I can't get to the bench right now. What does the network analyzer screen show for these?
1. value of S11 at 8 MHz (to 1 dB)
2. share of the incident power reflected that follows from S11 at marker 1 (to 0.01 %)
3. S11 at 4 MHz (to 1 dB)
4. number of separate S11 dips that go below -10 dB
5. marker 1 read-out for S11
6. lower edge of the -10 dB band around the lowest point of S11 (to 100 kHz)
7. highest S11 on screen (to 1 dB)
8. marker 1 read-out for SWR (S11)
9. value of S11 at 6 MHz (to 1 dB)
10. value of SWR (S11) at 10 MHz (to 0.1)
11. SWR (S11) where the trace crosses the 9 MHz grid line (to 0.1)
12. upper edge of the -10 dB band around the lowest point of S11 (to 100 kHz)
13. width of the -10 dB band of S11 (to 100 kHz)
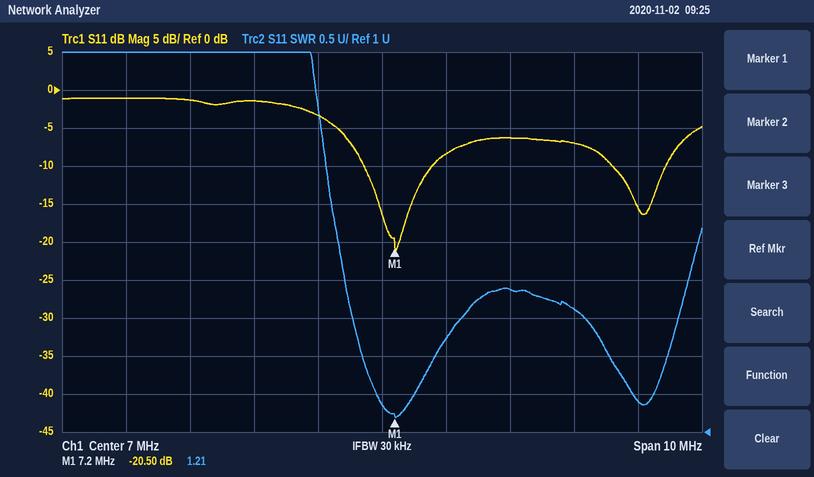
-8 dB
0.89 %
-1 dB
2
-20.50 dB
6.7 MHz
-1 dB
1.21
-3 dB
2.6
2.9
7.8 MHz
1.1 MHz
